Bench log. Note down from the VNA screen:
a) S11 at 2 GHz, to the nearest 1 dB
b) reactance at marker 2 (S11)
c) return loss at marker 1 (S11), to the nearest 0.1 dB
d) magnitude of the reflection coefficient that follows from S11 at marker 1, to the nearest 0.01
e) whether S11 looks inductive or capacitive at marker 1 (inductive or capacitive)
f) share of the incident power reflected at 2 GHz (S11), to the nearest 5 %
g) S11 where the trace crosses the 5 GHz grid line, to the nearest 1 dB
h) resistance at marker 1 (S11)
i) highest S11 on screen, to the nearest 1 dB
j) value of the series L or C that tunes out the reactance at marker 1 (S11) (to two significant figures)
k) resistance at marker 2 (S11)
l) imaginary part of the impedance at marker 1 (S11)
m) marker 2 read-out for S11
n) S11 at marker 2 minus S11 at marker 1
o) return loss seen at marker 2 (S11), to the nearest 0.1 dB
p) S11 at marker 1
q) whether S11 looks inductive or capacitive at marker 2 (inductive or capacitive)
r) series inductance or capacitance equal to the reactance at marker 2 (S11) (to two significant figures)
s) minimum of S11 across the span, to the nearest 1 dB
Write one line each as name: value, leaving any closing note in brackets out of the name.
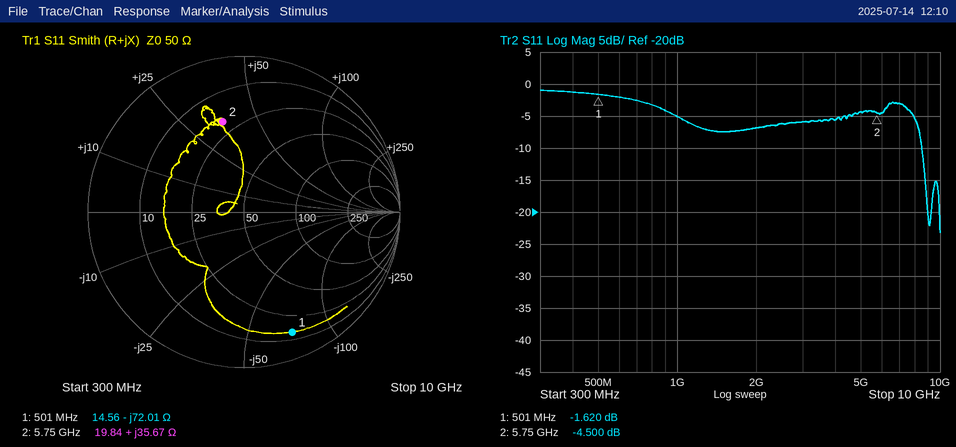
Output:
S11 at 2 GHz, to the nearest 1 dB: -7 dB
reactance at marker 2: +35.67 Ω
return loss at marker 1 (S11), to the nearest 0.1 dB: 1.6 dB
magnitude of the reflection coefficient that follows from S11 at marker 1, to the nearest 0.01: 0.83
whether S11 looks inductive or capacitive at marker 1: capacitive
share of the incident power reflected at 2 GHz (S11), to the nearest 5 %: 20 %
S11 where the trace crosses the 5 GHz grid line, to the nearest 1 dB: -4 dB
resistance at marker 1: 14.56 Ω
highest S11 on screen, to the nearest 1 dB: -1 dB
value of the series L or C that tunes out the reactance at marker 1 (S11): 23 nH
resistance at marker 2: 19.84 Ω
imaginary part of the impedance at marker 1: -72.01 Ω
marker 2 read-out for S11: -4.500 dB
S11 at marker 2 minus S11 at marker 1: -2.880 dB
return loss seen at marker 2 (S11), to the nearest 0.1 dB: 4.5 dB
S11 at marker 1: -1.620 dB
whether S11 looks inductive or capacitive at marker 2: inductive
series inductance or capacitance equal to the reactance at marker 2 (S11): 990 pH
minimum of S11 across the span, to the nearest 1 dB: -23 dB
